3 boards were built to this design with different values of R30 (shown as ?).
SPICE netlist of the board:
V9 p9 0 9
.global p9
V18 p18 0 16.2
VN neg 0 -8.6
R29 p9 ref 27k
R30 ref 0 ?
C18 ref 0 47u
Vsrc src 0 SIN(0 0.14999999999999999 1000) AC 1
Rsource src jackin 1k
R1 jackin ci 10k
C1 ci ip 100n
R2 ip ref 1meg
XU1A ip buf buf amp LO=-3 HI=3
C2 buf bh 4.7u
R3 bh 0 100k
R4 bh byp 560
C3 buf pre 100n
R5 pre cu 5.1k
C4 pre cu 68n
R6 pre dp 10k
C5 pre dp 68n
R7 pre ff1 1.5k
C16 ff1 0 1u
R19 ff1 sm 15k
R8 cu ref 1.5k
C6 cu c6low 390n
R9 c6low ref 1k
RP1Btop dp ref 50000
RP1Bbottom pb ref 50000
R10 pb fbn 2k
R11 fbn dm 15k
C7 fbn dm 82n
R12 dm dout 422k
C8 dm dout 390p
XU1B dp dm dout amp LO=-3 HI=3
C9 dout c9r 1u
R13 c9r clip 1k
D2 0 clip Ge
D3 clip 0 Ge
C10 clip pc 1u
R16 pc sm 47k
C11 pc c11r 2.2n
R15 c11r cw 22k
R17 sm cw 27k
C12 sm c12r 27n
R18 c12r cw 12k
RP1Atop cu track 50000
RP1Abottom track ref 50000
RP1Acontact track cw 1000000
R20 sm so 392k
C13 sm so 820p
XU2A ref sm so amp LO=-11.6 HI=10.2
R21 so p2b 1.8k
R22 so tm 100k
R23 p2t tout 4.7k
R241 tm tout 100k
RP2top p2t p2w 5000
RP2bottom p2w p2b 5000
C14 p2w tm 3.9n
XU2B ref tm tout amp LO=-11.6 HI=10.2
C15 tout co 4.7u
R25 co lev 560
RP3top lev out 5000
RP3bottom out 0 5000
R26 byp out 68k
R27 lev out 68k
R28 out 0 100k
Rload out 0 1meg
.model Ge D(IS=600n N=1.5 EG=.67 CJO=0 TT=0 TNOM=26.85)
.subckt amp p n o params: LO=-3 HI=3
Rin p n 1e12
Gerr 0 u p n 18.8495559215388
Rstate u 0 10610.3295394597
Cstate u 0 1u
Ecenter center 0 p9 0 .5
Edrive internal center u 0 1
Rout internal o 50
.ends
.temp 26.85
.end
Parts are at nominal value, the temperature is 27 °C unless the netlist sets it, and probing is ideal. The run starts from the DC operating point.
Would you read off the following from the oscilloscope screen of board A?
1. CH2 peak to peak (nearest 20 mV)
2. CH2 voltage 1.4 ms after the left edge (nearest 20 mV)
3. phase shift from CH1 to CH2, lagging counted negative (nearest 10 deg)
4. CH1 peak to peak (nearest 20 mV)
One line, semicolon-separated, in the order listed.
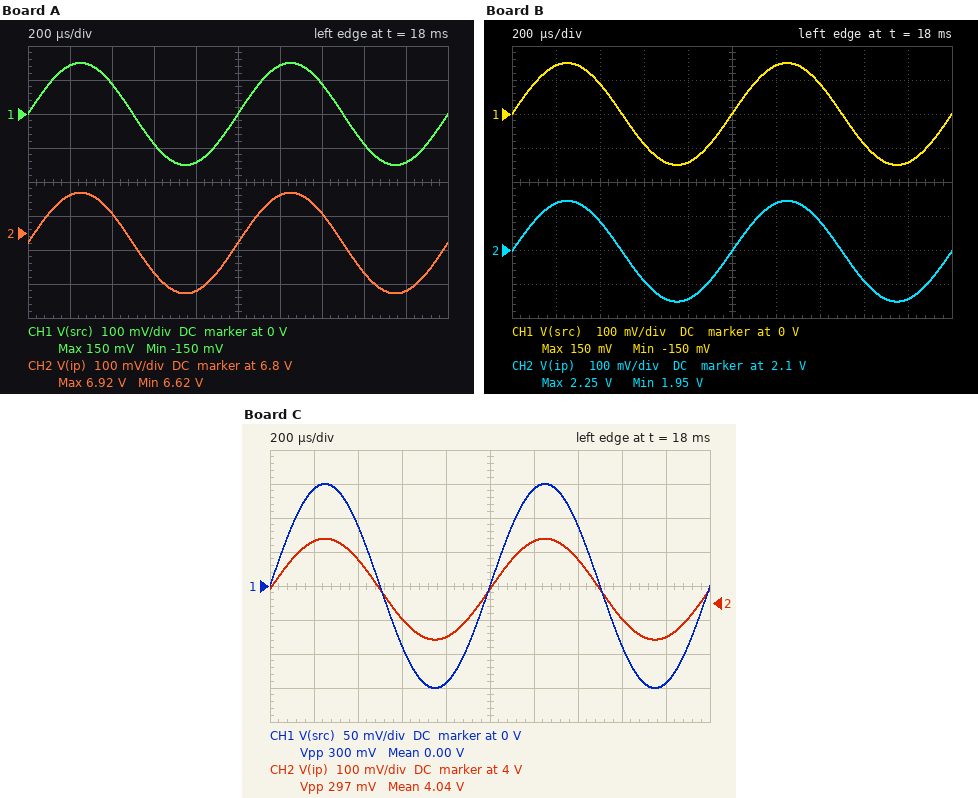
300 mV; 6.86 V; 0 deg; 300 mV
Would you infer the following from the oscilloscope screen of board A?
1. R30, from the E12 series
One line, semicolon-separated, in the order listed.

82 kΩ
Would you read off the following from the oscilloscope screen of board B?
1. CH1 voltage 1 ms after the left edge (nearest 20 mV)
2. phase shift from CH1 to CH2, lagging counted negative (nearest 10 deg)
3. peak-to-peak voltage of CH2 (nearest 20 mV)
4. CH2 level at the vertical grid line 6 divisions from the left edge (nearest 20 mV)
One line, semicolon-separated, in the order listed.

0 V; 0 deg; 300 mV; 2.24 V
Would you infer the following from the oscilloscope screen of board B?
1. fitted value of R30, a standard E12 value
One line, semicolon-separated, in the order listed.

8.2 kΩ
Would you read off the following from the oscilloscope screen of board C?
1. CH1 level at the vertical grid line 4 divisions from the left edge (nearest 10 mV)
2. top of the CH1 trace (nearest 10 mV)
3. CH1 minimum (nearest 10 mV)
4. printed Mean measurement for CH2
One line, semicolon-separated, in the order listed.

-140 mV; 150 mV; -150 mV; 4.04 V
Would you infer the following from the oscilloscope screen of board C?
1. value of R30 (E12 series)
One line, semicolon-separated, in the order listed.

22 kΩ
